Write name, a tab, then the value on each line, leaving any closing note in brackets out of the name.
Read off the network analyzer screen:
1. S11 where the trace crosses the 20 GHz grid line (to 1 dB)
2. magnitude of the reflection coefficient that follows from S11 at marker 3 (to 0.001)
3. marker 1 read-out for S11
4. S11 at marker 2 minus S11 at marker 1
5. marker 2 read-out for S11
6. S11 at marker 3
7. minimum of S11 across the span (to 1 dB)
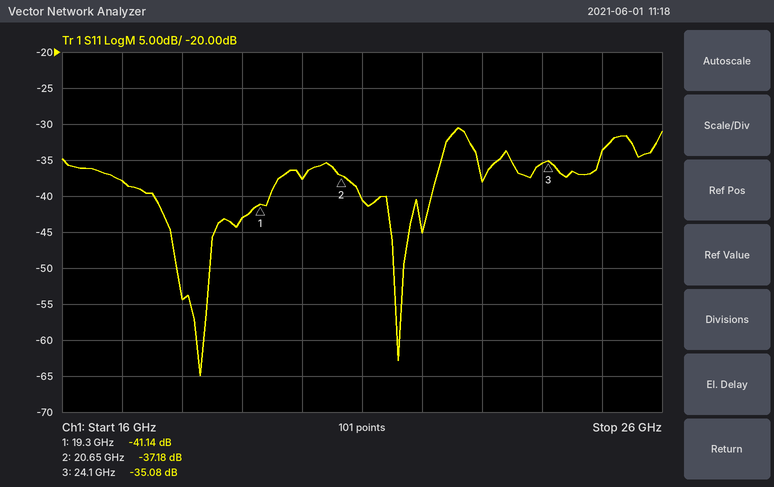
S11 where the trace crosses the 20 GHz grid line	-38 dB
magnitude of the reflection coefficient that follows from S11 at marker 3	0.018
marker 1 read-out for S11	-41.14 dB
S11 at marker 2 minus S11 at marker 1	3.96 dB
marker 2 read-out for S11	-37.18 dB
S11 at marker 3	-35.08 dB
minimum of S11 across the span	-65 dB
